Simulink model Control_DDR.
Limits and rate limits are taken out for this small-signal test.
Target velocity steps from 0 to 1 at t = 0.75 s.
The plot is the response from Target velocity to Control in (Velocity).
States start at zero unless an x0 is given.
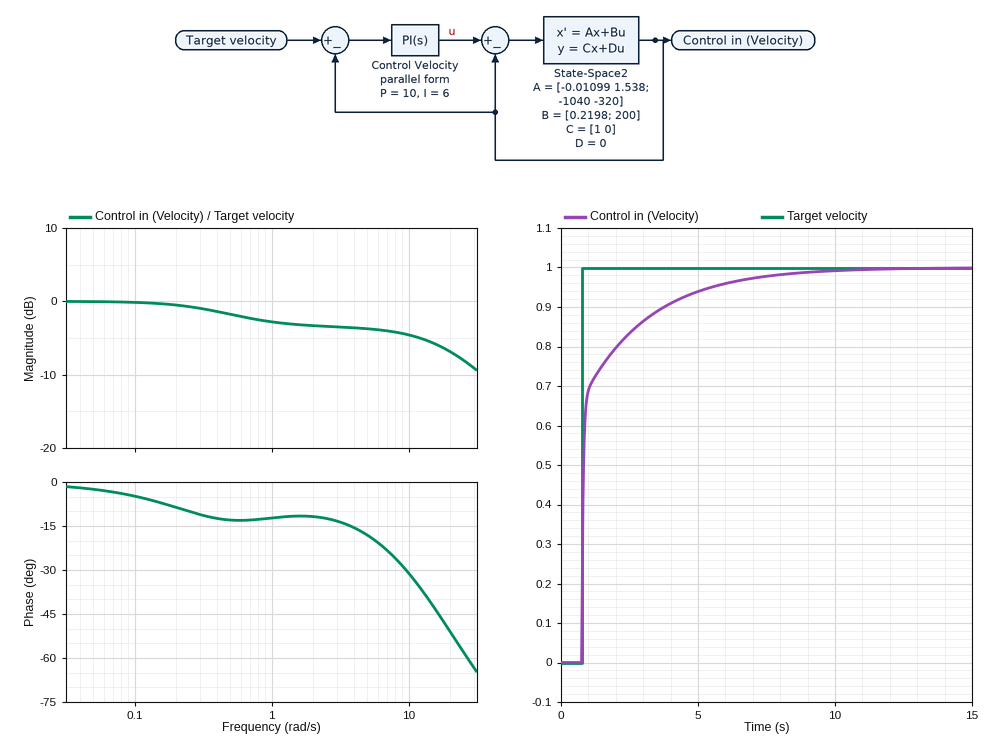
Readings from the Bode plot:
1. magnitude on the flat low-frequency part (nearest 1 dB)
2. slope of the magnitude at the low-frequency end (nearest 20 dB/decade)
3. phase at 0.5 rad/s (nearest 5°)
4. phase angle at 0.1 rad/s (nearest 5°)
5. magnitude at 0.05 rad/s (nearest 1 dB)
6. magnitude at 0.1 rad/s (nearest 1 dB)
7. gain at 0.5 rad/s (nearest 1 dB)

0 dB
0 dB/decade
-15°
-5°
0 dB
0 dB
-2 dB
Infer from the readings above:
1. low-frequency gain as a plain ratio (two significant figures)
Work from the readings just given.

1.0
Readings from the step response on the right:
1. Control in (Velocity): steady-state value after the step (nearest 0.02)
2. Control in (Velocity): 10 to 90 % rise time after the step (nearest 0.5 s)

1.00
3.0 s
